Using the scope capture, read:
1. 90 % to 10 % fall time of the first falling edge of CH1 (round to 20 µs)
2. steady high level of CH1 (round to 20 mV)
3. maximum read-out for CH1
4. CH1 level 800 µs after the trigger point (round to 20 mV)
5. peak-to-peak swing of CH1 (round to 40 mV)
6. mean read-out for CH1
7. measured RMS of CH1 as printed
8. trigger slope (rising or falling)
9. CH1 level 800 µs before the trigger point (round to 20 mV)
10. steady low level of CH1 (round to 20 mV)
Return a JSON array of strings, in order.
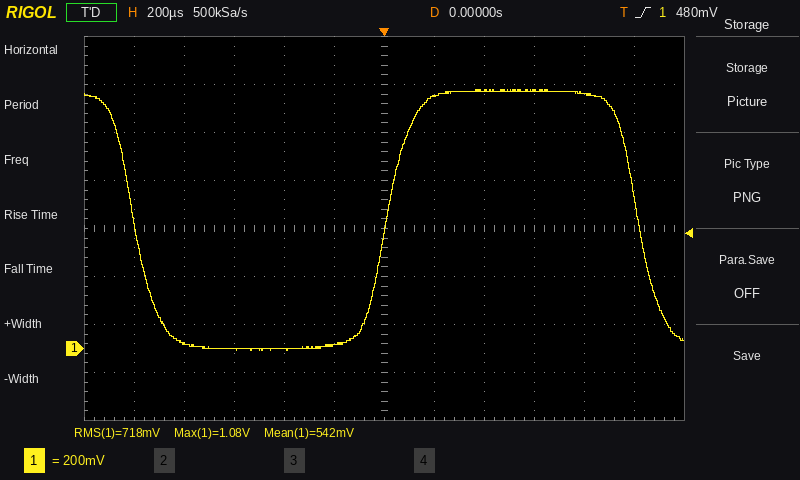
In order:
["200 µs", "1.08 V", "1.08 V", "1.06 V", "1.08 V", "542 mV", "718 mV", "rising", "20 mV", "0 mV"]
